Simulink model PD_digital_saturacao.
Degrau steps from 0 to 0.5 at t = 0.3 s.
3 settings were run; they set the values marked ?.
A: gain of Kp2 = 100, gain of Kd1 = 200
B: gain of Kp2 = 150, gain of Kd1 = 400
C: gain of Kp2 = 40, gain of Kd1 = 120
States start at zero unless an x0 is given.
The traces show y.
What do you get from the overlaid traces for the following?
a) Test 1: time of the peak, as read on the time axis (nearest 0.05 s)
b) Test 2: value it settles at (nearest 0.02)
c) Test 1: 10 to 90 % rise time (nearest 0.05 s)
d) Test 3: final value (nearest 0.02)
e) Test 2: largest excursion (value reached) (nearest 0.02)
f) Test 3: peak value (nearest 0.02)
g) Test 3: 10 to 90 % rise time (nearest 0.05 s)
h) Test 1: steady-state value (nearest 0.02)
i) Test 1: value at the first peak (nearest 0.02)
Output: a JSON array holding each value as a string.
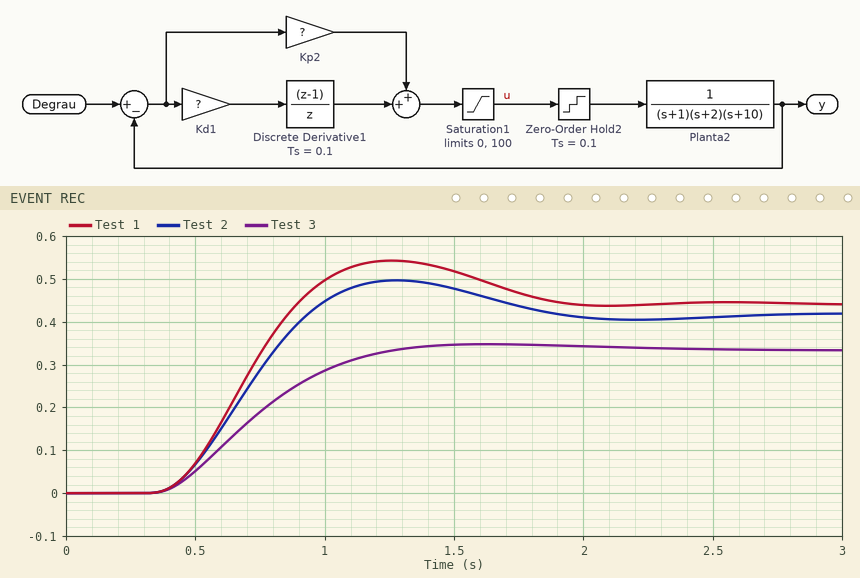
["1.25 s", "0.42", "0.35 s", "0.34", "0.50", "0.34", "0.60 s", "0.44", "0.54"]
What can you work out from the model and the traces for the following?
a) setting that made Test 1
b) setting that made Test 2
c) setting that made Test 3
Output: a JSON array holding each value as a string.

["B", "A", "C"]
